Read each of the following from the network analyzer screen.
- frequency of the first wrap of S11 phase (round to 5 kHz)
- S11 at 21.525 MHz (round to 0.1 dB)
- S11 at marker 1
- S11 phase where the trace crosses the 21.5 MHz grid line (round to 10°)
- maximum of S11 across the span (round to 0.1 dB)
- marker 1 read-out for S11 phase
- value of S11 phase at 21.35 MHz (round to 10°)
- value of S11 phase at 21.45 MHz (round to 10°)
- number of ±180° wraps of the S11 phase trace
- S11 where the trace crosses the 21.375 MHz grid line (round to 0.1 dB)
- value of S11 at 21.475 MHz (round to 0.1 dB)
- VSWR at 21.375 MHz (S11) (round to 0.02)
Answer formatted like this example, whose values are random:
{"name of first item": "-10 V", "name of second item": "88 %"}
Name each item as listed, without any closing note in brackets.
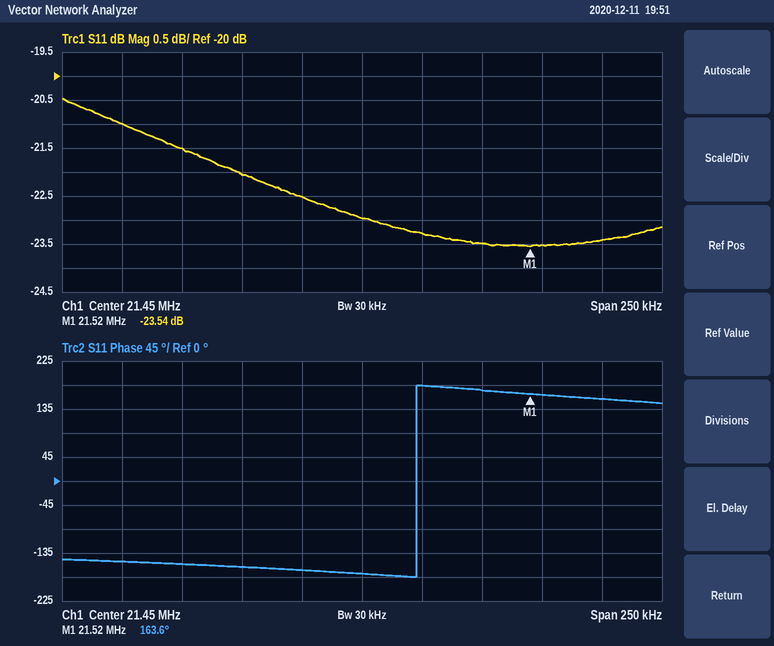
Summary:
{"frequency of the first wrap of S11 phase": "21.475 MHz", "S11 at 21.525 MHz": "-23.5 dB", "S11 at marker 1": "-23.54 dB", "S11 phase where the trace crosses the 21.5 MHz grid line": "170°", "maximum of S11 across the span": "-20.5 dB", "marker 1 read-out for S11 phase": "163.6°", "value of S11 phase at 21.35 MHz": "-150°", "value of S11 phase at 21.45 MHz": "-170°", "number of ±180° wraps of the S11 phase trace": "1", "S11 where the trace crosses the 21.375 MHz grid line": "-21.5 dB", "value of S11 at 21.475 MHz": "-23.3 dB", "VSWR at 21.375 MHz (S11)": "1.18"}
